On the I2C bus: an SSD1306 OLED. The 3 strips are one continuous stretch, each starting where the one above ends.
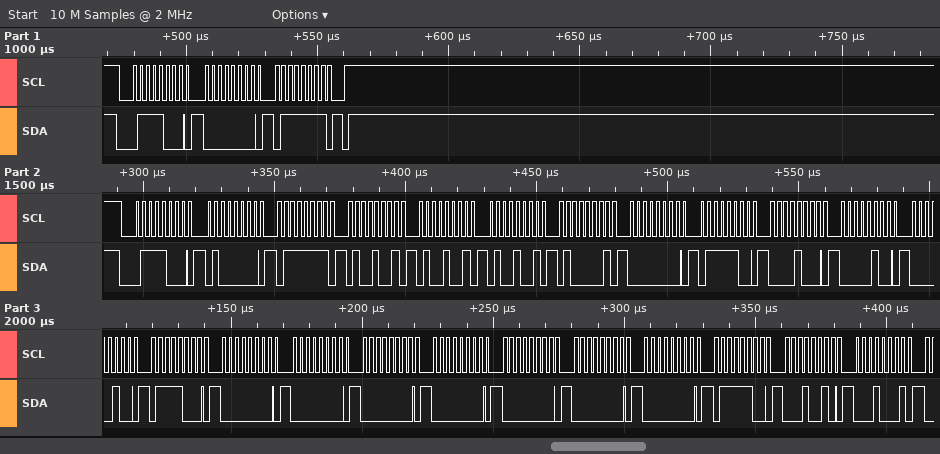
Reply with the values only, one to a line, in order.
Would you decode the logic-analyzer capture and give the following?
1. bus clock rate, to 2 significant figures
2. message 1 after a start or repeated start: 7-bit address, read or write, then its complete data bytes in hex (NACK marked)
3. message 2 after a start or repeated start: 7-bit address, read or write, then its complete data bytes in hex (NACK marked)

400 kHz
0x3C write: 00 7F
0x3C write: 40 7F 49 49 49 41 00 7C 08 04 04 78 00 00 00 00 00 00 00 7C 12 11
